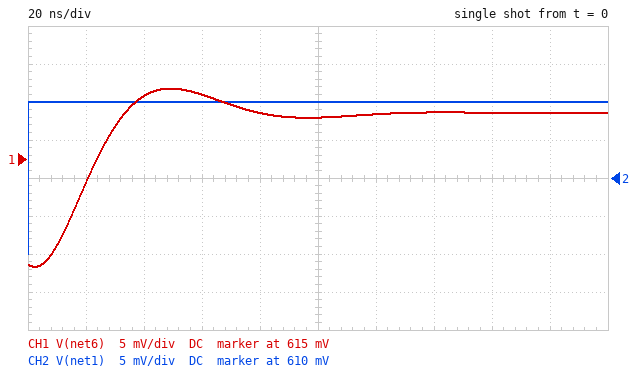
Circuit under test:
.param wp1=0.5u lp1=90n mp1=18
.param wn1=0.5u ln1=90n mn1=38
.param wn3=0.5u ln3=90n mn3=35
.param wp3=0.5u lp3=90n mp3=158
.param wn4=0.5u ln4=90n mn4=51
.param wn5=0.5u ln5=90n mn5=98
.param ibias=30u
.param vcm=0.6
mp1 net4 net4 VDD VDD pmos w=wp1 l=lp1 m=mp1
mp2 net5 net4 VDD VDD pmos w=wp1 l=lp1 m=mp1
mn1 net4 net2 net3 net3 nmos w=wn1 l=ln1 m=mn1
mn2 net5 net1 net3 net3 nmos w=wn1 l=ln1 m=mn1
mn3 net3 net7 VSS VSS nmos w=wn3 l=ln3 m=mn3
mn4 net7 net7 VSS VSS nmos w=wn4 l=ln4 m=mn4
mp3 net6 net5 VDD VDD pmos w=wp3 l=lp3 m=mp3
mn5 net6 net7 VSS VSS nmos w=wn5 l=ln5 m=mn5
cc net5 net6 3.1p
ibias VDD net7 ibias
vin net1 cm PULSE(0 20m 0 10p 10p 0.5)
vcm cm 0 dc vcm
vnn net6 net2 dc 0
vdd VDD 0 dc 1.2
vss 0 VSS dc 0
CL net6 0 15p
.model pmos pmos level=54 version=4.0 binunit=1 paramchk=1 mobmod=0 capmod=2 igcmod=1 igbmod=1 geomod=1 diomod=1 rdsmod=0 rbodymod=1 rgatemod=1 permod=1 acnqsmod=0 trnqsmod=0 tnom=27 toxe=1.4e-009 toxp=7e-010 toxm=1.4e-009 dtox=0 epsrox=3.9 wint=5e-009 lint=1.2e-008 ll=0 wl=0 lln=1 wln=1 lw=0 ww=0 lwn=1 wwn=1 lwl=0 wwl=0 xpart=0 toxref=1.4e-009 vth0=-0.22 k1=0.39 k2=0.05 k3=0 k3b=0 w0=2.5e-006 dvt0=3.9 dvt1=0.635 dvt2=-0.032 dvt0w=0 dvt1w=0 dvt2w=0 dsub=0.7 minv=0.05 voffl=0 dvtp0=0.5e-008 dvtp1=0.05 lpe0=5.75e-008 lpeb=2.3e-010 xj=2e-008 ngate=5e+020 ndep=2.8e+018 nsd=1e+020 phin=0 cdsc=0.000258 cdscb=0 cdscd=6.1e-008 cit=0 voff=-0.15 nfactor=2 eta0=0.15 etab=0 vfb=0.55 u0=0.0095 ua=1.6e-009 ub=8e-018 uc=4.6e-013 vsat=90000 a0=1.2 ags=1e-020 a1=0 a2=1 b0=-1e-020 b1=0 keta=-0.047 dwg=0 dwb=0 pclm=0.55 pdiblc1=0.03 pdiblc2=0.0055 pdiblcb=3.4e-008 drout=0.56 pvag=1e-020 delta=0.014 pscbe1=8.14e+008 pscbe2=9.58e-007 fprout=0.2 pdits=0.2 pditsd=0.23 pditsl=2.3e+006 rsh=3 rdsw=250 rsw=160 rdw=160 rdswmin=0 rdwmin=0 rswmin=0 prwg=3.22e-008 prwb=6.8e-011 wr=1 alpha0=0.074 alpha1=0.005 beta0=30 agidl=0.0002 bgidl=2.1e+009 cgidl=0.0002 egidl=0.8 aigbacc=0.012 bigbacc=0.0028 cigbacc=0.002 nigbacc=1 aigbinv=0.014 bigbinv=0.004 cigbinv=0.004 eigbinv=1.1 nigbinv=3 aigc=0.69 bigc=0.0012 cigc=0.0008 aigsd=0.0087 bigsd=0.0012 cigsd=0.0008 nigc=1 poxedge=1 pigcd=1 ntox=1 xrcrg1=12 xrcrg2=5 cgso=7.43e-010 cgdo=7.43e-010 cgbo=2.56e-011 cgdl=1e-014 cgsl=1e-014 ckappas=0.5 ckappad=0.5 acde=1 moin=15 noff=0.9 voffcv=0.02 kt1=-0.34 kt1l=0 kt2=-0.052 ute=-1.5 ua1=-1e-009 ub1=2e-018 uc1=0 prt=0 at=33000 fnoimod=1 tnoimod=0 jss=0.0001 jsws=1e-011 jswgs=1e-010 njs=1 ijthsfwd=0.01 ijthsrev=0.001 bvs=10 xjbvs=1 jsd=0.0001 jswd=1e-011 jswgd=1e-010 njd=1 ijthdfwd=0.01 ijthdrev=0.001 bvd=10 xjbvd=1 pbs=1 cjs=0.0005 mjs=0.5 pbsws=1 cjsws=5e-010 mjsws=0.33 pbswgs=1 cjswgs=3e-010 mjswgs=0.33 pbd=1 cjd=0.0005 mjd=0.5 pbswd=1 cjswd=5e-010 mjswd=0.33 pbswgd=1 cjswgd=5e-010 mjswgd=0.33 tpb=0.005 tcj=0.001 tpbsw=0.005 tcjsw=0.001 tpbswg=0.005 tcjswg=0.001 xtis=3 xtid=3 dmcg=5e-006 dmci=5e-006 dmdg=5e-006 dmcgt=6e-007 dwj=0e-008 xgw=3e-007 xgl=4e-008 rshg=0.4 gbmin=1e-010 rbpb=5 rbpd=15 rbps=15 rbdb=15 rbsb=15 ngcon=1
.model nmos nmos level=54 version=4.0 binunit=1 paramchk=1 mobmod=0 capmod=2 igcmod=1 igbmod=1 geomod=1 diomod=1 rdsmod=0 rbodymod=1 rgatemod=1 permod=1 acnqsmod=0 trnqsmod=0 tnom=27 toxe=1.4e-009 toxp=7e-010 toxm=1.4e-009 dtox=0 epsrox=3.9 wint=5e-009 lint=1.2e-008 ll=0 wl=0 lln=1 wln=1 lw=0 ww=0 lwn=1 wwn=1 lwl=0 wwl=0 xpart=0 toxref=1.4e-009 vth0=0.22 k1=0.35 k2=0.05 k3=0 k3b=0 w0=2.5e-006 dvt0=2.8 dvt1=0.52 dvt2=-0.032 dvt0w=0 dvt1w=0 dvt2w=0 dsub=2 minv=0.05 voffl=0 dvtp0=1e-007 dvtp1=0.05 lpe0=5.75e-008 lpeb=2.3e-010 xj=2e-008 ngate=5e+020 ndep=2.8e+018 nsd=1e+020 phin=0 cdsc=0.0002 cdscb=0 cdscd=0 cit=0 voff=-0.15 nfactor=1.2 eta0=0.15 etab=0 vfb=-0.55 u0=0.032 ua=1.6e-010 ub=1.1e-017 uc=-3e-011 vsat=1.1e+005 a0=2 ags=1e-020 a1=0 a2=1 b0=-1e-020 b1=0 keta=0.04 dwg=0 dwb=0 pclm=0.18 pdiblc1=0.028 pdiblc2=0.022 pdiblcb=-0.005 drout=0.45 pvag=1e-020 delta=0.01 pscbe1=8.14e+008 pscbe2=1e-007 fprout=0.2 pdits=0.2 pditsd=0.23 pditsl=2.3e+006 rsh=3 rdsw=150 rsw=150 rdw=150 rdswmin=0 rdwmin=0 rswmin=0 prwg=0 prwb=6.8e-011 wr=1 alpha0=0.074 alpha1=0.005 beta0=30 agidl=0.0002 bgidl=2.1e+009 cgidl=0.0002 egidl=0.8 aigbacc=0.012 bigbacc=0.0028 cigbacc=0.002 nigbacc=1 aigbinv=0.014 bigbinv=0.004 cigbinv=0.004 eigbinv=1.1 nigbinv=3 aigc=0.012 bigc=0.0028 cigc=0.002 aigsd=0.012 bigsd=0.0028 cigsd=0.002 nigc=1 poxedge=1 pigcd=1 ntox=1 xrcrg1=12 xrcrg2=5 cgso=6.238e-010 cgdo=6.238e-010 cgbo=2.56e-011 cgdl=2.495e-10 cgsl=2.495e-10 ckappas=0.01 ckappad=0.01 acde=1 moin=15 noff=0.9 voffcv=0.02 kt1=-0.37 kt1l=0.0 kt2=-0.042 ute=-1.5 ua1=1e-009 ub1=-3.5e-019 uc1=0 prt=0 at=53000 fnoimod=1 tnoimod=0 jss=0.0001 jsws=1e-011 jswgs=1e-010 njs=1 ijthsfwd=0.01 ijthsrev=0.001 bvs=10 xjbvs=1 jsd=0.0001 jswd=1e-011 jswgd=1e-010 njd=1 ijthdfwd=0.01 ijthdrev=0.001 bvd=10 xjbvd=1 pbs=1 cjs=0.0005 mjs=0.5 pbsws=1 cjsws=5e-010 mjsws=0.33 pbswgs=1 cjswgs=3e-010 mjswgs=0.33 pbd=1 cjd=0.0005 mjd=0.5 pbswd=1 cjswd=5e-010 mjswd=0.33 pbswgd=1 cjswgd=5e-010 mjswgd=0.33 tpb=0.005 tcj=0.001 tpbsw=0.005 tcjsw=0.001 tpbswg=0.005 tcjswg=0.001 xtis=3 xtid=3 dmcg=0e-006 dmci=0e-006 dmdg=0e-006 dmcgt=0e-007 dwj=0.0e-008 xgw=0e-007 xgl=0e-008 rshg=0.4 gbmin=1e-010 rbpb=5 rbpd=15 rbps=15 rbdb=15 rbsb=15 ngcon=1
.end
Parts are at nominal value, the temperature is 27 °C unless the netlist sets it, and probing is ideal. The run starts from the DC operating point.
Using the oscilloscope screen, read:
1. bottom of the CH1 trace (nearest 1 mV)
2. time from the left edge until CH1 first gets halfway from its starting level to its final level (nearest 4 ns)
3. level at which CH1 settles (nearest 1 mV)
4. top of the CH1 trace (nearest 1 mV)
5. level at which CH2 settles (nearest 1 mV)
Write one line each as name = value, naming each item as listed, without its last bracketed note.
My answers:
bottom of the CH1 trace = 601 mV
time from the left edge until CH1 first gets halfway from its starting level to its final level = 20 ns
level at which CH1 settles = 621 mV
top of the CH1 trace = 624 mV
level at which CH2 settles = 620 mV
